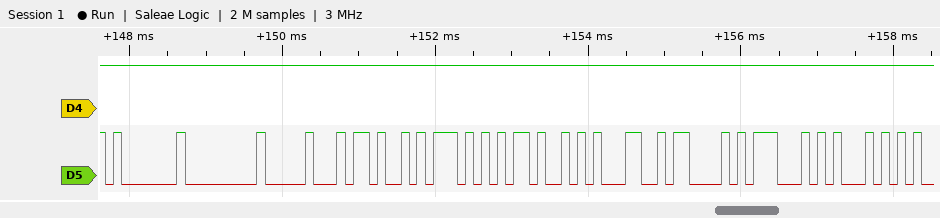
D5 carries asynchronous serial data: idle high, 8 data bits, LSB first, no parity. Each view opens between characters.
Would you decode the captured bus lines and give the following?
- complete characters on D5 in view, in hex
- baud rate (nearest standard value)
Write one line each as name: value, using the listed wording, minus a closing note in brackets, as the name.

complete characters on D5 in view, in hex: 01, 00, 10, 4B, 57, 4B, 31, 43, 47, 51
baud rate: 9600 baud
